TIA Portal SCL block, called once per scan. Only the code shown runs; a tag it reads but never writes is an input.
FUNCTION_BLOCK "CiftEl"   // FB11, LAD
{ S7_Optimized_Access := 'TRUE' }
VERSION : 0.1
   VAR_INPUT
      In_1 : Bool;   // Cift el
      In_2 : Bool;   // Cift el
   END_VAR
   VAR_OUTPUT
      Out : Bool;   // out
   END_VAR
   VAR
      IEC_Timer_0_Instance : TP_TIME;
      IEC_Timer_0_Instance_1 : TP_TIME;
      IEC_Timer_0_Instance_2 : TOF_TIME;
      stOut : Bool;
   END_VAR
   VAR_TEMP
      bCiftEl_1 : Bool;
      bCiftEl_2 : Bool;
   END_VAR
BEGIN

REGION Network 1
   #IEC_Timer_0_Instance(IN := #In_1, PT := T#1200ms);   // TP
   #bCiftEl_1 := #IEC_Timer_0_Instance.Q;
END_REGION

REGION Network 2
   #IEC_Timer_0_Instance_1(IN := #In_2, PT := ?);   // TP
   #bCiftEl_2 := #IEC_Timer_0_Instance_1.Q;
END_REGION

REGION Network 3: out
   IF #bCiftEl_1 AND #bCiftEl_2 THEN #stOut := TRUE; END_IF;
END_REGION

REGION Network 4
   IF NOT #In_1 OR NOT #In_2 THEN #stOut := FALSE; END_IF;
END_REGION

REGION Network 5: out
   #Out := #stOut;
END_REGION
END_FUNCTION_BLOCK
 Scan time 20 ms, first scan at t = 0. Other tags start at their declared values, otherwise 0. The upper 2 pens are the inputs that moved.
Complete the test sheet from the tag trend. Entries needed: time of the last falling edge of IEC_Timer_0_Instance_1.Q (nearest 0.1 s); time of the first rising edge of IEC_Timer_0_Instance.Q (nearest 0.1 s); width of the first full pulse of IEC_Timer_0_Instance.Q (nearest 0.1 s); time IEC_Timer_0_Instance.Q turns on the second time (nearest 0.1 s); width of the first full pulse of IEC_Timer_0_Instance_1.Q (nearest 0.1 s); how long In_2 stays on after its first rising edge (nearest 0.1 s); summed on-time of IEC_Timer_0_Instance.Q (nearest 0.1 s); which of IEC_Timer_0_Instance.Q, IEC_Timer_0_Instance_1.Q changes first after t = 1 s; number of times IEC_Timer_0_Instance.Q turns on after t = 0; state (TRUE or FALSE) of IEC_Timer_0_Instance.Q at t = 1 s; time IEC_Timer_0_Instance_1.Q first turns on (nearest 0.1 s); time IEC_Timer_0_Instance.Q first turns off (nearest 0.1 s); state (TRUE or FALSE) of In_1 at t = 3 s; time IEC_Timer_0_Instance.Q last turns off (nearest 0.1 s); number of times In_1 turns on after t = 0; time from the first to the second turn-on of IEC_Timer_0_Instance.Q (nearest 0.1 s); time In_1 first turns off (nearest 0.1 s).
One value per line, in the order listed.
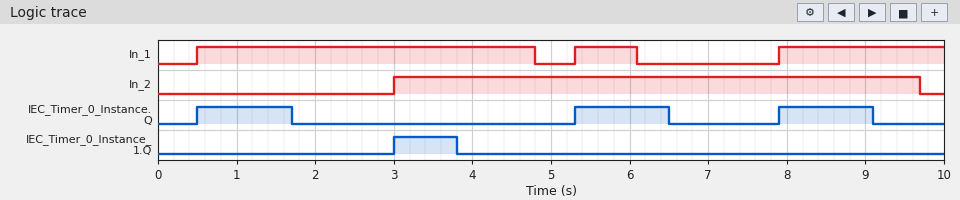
3.8 s
0.5 s
1.2 s
5.3 s
0.8 s
6.7 s
3.6 s
IEC_Timer_0_Instance.Q
3
TRUE
3.0 s
1.7 s
TRUE
9.1 s
3
4.8 s
4.8 s
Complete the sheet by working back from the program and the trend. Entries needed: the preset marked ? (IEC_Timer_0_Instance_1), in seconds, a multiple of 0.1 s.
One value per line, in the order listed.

0.8 s
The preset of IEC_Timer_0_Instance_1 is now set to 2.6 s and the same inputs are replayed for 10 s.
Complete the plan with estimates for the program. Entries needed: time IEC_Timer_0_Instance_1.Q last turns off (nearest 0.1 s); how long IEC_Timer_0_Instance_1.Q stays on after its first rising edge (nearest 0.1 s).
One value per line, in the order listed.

5.6 s
2.6 s
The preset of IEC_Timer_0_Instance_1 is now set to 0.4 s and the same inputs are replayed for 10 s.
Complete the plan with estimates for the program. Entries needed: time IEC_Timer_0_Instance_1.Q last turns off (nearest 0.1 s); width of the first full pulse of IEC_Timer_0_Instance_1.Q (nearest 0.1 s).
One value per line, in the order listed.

3.4 s
0.4 s
